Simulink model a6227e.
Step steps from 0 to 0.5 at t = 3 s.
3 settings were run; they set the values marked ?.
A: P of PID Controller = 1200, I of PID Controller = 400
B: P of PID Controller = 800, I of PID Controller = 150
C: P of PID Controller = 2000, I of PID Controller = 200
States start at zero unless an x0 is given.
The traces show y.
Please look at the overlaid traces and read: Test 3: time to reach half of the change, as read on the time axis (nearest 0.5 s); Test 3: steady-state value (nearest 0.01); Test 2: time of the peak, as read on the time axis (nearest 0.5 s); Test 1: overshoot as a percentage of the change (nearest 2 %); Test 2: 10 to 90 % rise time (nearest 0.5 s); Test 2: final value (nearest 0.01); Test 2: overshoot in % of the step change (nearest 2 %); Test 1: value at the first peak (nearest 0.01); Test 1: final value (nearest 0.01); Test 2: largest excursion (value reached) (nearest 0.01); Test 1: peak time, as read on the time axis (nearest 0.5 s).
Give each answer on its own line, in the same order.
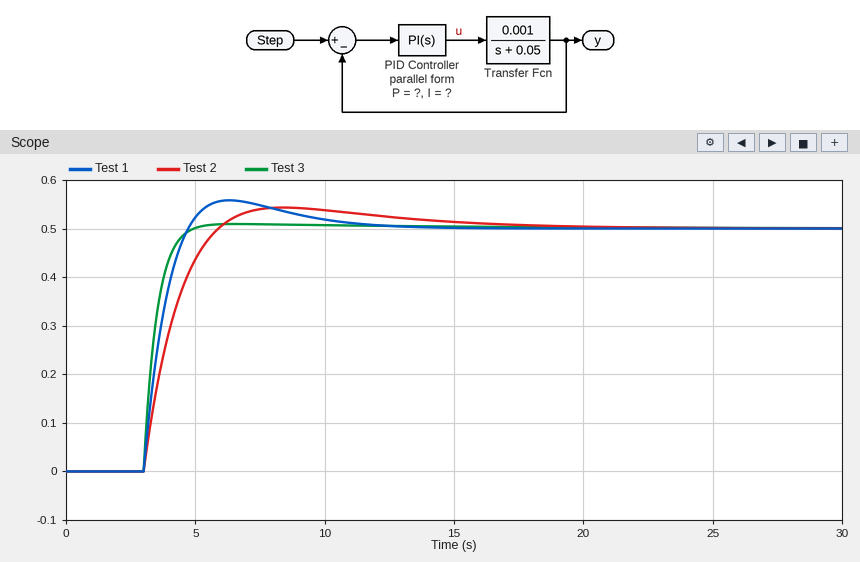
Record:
3.5 s
0.50
8.5 s
12 %
2.0 s
0.50
8 %
0.56
0.50
0.54
6.5 s
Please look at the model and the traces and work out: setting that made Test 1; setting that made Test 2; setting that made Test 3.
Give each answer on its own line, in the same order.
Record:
A
B
C
